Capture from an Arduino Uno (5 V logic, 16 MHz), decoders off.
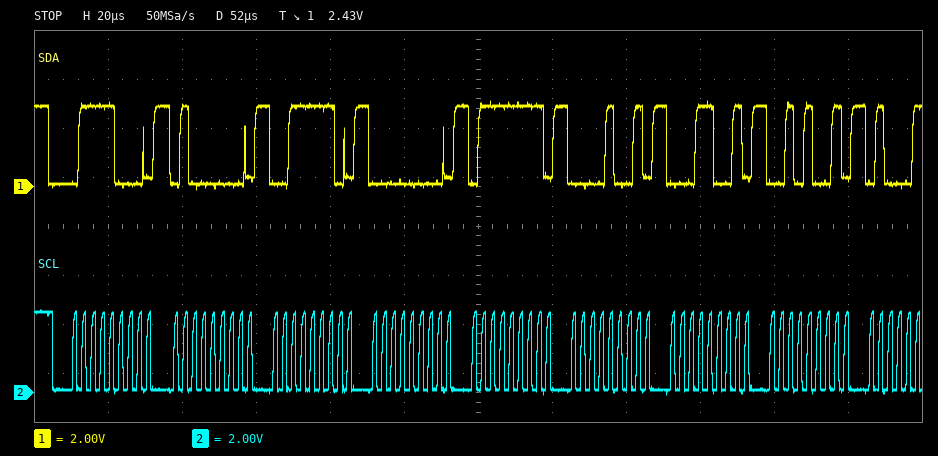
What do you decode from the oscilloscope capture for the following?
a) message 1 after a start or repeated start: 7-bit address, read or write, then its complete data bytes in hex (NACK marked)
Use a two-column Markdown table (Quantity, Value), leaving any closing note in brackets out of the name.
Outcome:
| Quantity | Value |
|---|---|
| message 1 after a start or repeated start: 7-bit address, read or write, then its complete data bytes in hex | 0x3C write: 40 3E 00 7F 09 19 29 |
